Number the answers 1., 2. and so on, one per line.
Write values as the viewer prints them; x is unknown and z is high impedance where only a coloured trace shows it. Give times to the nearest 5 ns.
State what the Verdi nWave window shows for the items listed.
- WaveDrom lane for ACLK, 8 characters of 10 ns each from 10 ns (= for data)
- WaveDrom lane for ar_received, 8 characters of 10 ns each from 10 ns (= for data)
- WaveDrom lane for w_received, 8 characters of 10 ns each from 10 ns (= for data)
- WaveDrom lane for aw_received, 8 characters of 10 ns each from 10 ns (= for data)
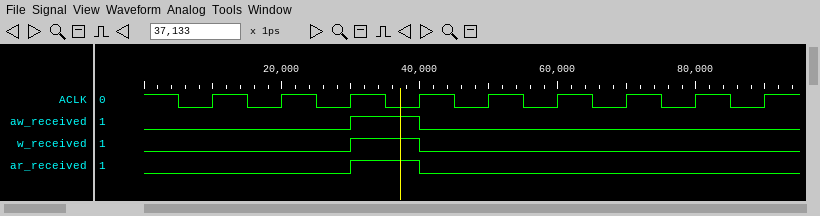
1. {name: 'ACLK', wave: 'p.......'}
2. {name: 'ar_received', wave: '0.10....'}
3. {name: 'w_received', wave: '0.10....'}
4. {name: 'aw_received', wave: '0.10....'}
